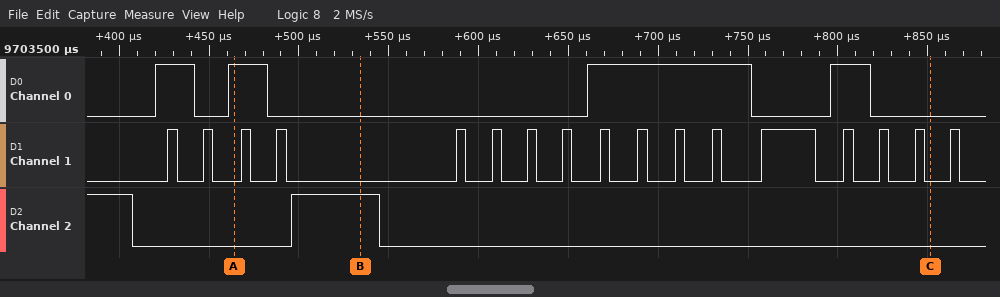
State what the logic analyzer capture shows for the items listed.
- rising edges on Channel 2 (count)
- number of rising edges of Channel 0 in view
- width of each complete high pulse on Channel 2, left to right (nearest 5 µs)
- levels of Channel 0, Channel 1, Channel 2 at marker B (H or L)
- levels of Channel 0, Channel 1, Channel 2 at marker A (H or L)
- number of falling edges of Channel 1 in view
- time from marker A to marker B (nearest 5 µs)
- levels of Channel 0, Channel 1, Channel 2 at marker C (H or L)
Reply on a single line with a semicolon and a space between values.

1; 4; 50 µs; Channel 0=L, Channel 1=L, Channel 2=H; Channel 0=H, Channel 1=L, Channel 2=L; 17; 70 µs; Channel 0=L, Channel 1=L, Channel 2=L
